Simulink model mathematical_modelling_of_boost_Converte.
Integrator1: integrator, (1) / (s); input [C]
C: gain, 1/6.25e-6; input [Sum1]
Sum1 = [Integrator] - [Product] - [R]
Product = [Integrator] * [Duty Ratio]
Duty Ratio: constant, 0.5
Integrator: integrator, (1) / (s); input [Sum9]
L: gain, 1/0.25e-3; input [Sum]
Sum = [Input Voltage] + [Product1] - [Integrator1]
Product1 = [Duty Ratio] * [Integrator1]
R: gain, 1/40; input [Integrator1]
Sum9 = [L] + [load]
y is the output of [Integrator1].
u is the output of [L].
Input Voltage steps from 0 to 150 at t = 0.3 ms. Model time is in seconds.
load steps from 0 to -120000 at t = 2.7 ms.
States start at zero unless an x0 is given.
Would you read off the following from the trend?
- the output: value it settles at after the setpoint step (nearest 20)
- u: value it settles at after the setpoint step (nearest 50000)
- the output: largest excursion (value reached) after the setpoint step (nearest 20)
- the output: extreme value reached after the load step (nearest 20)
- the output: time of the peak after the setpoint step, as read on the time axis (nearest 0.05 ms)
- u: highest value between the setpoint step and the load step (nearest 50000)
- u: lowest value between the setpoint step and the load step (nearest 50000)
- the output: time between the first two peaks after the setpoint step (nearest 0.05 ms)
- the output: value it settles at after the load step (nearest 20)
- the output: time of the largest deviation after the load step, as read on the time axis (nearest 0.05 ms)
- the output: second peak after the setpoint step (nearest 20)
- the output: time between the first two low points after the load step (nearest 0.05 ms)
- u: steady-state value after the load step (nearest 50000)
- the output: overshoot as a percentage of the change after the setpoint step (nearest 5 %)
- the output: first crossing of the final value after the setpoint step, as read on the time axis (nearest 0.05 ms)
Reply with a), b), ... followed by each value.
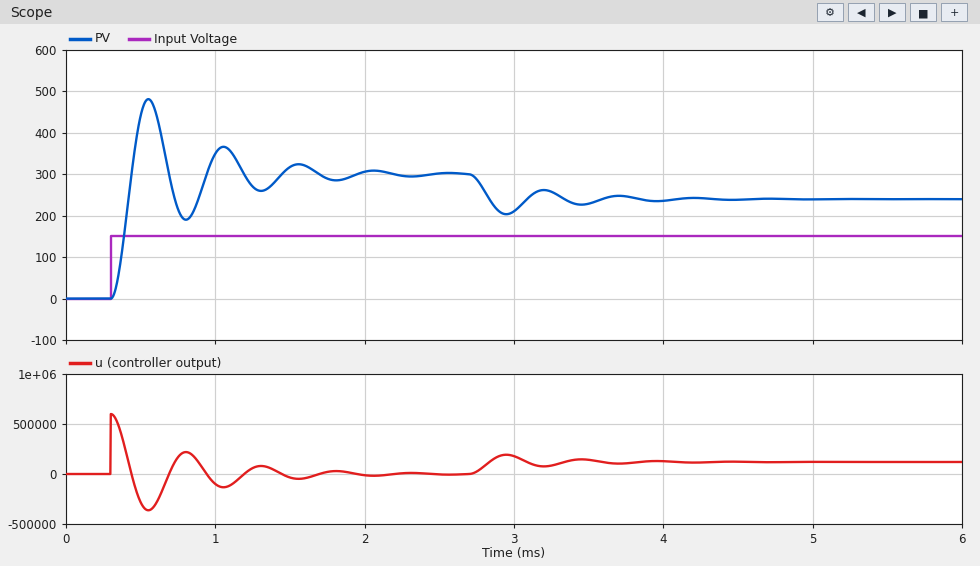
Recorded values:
a) 300
b) 0
c) 480
d) 200
e) 0.55 ms
f) 600000
g) -350000
h) 0.50 ms
i) 240
j) 2.95 ms
k) 360
l) 0.50 ms
m) 100000
n) 60 %
o) 0.45 ms
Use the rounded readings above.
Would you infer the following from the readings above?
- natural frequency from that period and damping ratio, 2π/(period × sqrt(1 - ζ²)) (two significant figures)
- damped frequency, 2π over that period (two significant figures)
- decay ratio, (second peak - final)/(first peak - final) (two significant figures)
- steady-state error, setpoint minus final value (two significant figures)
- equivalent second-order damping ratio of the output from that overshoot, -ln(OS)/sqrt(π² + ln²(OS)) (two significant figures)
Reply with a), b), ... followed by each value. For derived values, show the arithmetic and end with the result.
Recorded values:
a) 2π / (0.5 × sqrt(1 - 0.16²)) = 13 rad/ms
b) 2π / 0.5 = 13 rad/ms
c) (360 - 300) / (480 - 300) = 0.33
d) 150 - 300 = -150
e) ln(0.6) = -0.511; 0.511 / sqrt(9.870 + 0.261) = 0.16
